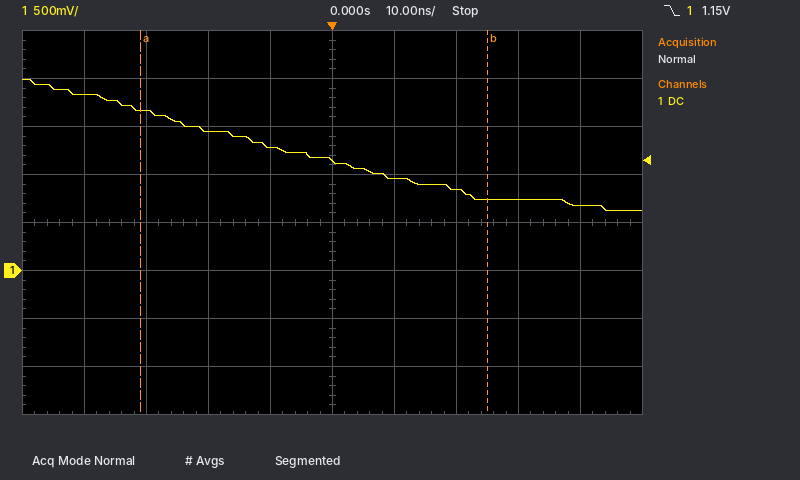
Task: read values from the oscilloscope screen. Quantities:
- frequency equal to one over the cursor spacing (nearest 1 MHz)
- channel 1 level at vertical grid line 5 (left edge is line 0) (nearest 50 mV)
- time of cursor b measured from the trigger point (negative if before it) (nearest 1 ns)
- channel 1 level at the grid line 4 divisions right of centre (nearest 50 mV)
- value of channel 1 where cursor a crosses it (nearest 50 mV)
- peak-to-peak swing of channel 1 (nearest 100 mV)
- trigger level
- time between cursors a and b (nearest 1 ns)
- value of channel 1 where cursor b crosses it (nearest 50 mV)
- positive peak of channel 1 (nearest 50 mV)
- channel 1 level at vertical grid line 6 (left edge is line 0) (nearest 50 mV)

18 MHz
1.15 V
+25 ns
700 mV
1.65 V
1.40 V
1.15 V
56 ns
750 mV
2.00 V
950 mV
